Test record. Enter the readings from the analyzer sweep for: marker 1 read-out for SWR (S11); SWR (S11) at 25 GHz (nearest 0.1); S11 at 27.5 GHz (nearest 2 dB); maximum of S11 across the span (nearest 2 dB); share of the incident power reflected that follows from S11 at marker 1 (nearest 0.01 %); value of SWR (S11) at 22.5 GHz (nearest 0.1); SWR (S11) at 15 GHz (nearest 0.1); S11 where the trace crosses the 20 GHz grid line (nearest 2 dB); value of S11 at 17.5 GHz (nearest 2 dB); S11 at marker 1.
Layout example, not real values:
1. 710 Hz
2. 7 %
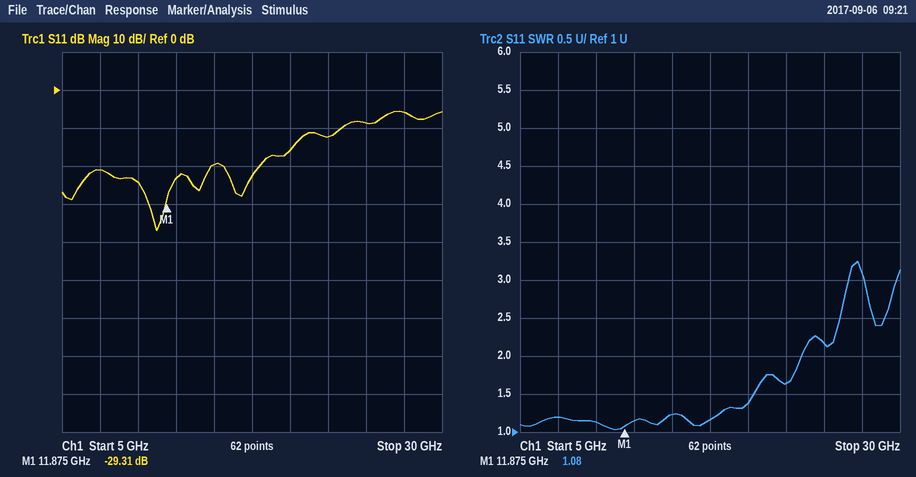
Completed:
1. 1.08
2. 2.2
3. -6 dB
4. -6 dB
5. 0.12 %
6. 1.6
7. 1.2
8. -16 dB
9. -22 dB
10. -29.31 dB
